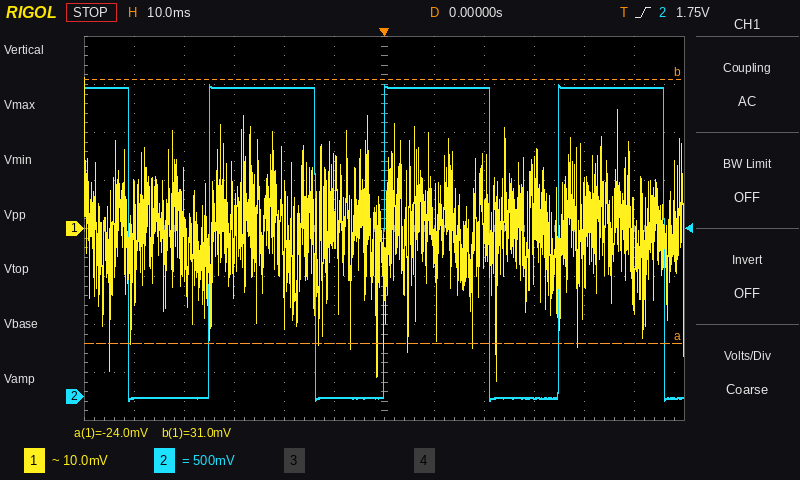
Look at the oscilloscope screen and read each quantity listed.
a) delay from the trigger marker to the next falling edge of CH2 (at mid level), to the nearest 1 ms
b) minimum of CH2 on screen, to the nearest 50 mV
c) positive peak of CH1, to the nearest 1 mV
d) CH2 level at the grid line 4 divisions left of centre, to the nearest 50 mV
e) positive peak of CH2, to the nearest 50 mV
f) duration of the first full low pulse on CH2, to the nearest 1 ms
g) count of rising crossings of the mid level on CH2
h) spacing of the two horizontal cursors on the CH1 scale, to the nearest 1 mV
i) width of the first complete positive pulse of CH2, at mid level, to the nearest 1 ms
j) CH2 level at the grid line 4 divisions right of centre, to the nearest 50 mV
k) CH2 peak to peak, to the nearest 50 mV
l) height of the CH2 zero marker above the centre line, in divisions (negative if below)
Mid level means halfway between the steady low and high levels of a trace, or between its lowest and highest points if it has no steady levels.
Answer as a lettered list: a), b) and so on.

a) 21 ms
b) -50 mV
c) 31 mV
d) 0 mV
e) 3.25 V
f) 16 ms
g) 3
h) 55 mV
i) 21 ms
j) 3.20 V
k) 3.30 V
l) -3.5 div
